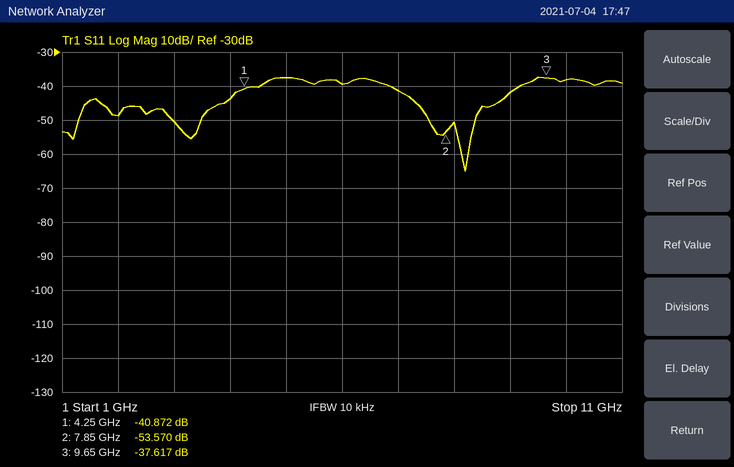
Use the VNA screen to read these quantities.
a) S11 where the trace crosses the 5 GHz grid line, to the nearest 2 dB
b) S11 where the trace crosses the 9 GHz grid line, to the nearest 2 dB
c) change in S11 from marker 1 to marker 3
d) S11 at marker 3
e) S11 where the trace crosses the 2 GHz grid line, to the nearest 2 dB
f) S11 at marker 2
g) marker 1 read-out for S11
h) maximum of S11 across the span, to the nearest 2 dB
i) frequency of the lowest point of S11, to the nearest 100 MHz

-38 dB
-42 dB
3.255 dB
-37.617 dB
-48 dB
-53.570 dB
-40.872 dB
-38 dB
8.2 GHz
